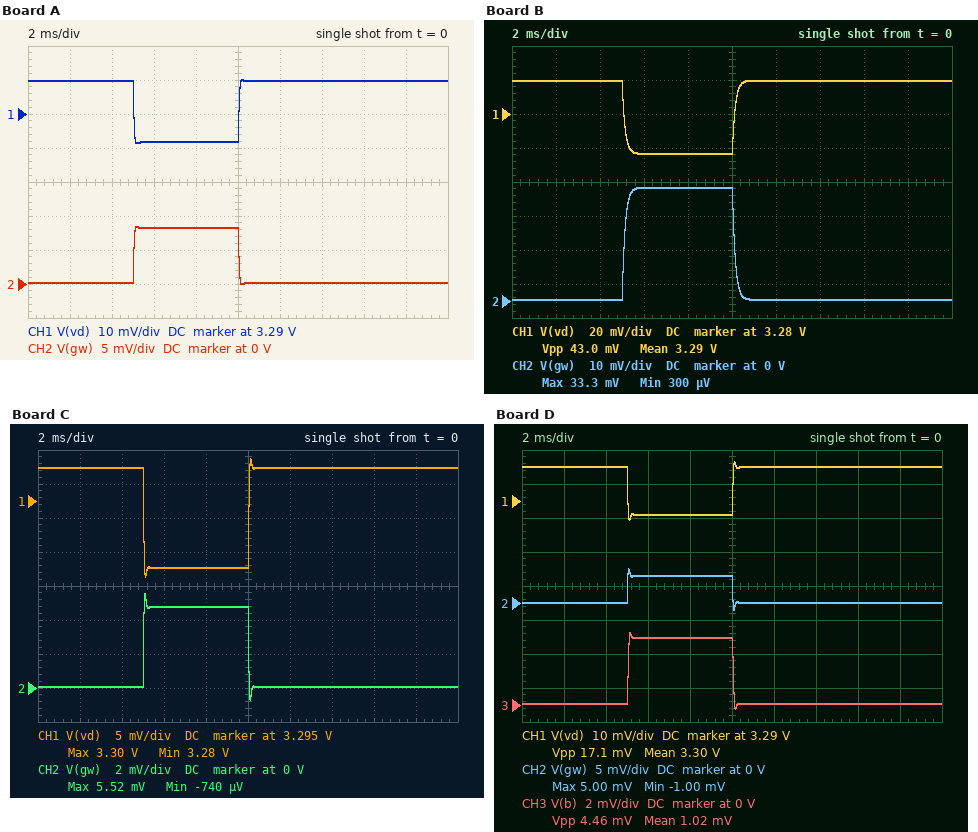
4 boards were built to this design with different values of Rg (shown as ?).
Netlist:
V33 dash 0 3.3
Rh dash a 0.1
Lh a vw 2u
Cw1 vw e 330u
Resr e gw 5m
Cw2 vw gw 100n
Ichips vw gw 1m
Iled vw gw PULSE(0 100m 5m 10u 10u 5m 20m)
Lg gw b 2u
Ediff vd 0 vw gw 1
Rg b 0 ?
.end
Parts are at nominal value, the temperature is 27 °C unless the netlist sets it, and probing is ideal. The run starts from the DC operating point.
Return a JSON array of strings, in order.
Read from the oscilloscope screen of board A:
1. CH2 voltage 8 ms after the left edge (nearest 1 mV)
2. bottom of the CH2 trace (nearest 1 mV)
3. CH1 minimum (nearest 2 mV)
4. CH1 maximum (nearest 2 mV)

["8 mV", "0 V", "3.282 V", "3.300 V"]
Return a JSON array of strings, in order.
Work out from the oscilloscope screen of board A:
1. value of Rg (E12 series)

["0.082 Ω"]
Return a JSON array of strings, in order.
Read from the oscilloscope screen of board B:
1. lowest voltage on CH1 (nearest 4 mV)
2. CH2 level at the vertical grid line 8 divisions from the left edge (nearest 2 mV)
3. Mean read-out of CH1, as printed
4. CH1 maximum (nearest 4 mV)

["3.256 V", "0 V", "3.29 V", "3.300 V"]
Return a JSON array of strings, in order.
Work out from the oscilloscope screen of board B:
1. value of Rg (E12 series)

["0.33 Ω"]
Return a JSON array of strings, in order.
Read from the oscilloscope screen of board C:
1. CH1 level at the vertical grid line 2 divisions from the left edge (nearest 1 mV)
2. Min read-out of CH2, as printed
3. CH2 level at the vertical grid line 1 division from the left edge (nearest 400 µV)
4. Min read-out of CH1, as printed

["3.300 V", "-740 µV", "0 V", "3.28 V"]
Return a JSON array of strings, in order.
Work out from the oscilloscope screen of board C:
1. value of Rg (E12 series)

["0.047 Ω"]
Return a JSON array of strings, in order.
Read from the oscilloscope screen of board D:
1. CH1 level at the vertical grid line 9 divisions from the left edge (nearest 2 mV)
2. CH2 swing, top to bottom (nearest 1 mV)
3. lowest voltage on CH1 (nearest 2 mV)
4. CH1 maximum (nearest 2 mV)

["3.300 V", "6 mV", "3.284 V", "3.302 V"]
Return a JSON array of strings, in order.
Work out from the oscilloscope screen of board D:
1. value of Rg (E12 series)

["0.039 Ω"]
